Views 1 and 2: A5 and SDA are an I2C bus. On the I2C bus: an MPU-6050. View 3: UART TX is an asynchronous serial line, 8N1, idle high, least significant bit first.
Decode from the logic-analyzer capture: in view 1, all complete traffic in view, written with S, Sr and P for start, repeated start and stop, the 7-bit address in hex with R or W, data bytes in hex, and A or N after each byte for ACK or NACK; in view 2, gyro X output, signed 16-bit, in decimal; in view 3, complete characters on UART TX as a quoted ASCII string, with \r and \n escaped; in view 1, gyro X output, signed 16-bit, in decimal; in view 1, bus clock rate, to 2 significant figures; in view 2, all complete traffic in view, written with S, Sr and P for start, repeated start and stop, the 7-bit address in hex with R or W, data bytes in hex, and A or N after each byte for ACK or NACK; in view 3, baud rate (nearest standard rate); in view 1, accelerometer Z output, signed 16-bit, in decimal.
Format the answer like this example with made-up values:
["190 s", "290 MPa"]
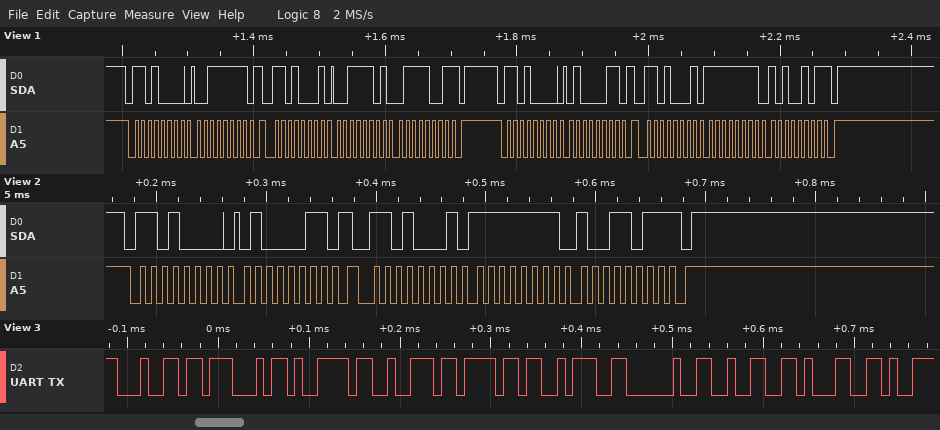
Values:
["S 68W A 3F A Sr 68R A 3D A 79 N P S 68W A 43 A Sr 68R A FF A A5 N P", "-101", "\"dGyro: 21\"", "-91", "100 kHz", "S 68W A 43 A Sr 68R A FF A 9B N P", "115200 baud", "15737"]
